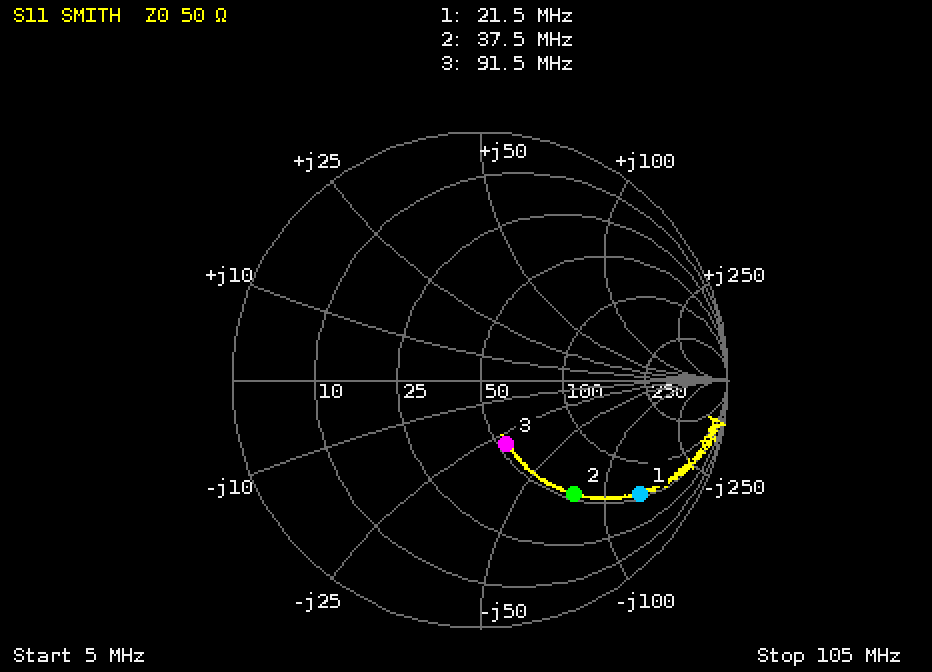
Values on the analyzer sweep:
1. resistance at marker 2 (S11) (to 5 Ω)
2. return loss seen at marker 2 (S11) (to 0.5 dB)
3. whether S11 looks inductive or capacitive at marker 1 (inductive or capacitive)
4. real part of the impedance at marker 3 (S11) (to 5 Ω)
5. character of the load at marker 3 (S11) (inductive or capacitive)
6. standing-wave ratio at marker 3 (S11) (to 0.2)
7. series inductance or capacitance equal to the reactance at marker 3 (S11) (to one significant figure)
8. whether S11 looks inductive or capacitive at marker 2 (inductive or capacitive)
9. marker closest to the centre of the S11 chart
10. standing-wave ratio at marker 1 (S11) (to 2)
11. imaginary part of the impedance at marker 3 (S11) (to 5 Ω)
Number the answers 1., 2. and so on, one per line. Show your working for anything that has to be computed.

1. 55 Ω
2. 4.5 dB
3. capacitive
4. 55 Ω
5. capacitive
6. 1.8
7. C = 1/(2π × 91.5 MHz × 30 Ω) ≈ 58.0 pF, so 60 pF to one significant figure
8. capacitive
9. marker 3
10. 8
11. -30 Ω
